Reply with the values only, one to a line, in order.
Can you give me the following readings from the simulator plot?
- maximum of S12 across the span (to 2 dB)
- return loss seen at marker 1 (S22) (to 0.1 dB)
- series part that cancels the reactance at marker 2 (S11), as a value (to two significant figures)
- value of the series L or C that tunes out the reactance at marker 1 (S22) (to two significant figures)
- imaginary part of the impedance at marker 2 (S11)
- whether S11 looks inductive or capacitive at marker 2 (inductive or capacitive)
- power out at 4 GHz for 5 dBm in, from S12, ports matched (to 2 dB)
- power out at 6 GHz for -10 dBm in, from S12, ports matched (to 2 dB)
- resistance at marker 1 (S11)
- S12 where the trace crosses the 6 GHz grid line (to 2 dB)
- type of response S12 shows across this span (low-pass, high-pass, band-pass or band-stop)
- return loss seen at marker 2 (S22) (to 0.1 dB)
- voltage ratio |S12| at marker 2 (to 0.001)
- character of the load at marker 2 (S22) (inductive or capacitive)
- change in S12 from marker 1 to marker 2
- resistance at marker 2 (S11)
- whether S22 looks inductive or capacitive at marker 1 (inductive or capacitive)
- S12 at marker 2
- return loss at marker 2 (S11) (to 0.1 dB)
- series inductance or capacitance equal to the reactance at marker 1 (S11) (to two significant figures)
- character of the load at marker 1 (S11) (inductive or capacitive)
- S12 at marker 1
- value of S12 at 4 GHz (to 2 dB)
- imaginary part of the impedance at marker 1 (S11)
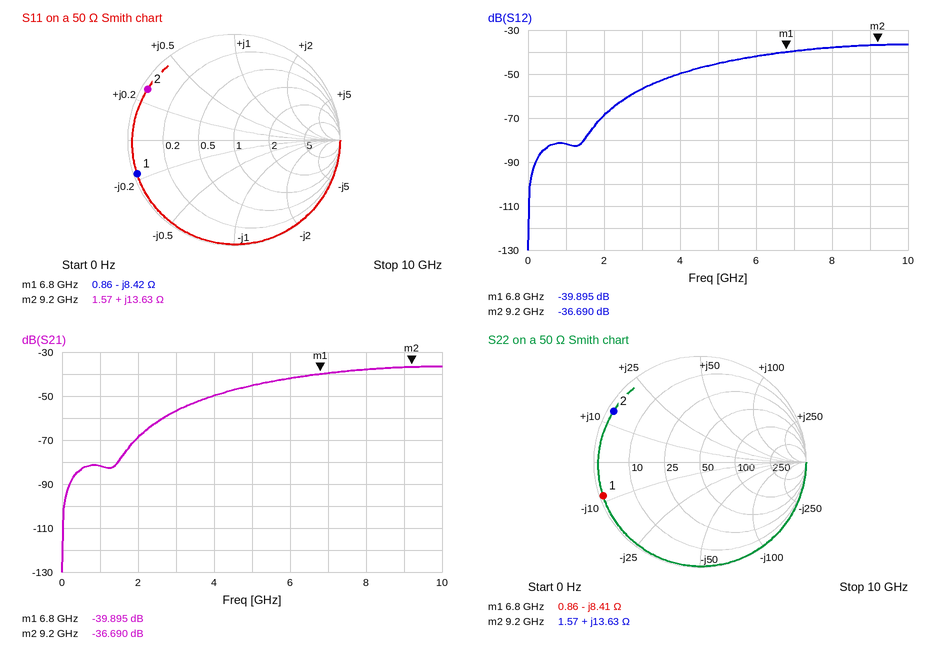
-36 dB
0.3 dB
1.3 pF
200 pH
+13.63 Ω
inductive
-44 dBm
-52 dBm
0.86 Ω
-42 dB
high-pass
0.5 dB
0.015
inductive
3.205 dB
1.57 Ω
capacitive
-36.690 dB
0.5 dB
2.8 pF
capacitive
-39.895 dB
-50 dB
-8.42 Ω
